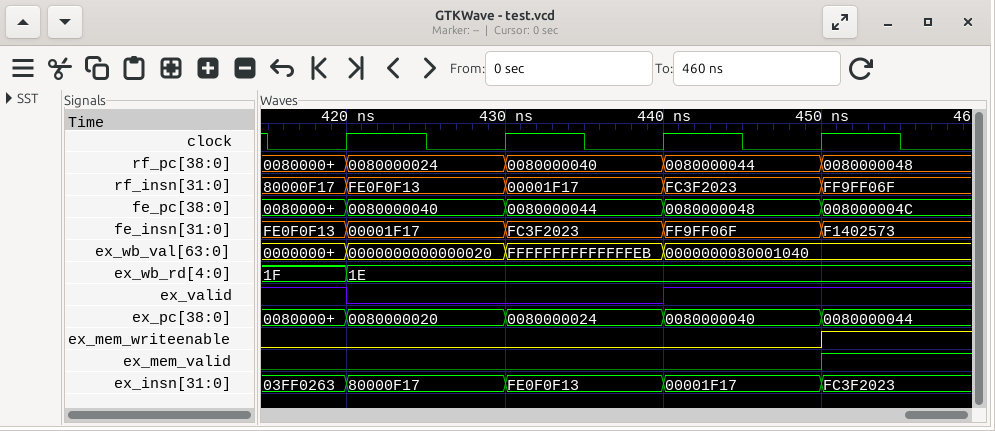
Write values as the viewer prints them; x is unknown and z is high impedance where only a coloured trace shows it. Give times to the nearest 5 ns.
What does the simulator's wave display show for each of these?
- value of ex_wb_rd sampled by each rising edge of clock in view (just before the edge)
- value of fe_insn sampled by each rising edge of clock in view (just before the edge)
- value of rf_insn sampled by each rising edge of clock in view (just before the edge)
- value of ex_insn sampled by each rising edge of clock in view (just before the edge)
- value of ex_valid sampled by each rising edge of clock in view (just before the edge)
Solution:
1F, 1E, 1E, 1E
FE0F0F13, 00001F17, FC3F2023, FF9FF06F
80000F17, FE0F0F13, 00001F17, FC3F2023
03FF0263, 80000F17, FE0F0F13, 00001F17
1 0 0 1
